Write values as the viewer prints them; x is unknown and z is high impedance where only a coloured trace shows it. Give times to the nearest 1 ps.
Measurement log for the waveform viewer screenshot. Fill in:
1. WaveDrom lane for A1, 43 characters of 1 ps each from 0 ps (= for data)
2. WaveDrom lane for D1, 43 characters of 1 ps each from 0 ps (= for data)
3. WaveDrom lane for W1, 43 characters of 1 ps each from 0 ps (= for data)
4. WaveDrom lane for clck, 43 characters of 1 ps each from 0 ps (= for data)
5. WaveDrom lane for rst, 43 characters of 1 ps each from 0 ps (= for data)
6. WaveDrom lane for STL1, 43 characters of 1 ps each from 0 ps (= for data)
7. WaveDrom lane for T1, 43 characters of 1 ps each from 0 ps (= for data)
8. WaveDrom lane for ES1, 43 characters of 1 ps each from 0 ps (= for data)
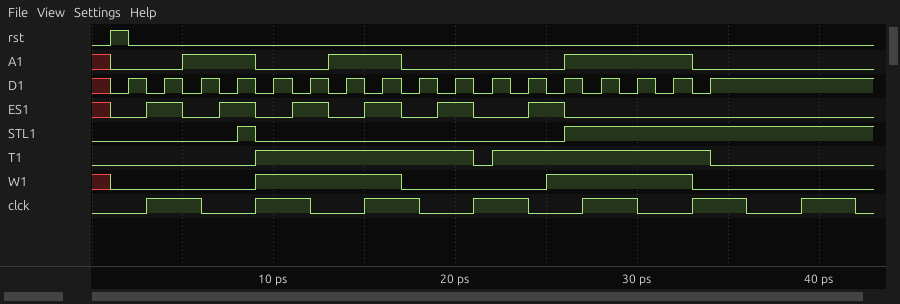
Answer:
{name: 'A1', wave: 'x0...1...0...1...0........1......0.........'}
{name: 'D1', wave: 'x0101010101010101010101010101010101........'}
{name: 'W1', wave: 'x0.......1.......0.......1.......0.........'}
{name: 'clck', wave: '0..1..0..1..0..1..0..1..0..1..0..1..0..1..0'}
{name: 'rst', wave: '010........................................'}
{name: 'STL1', wave: '0.......10................1................'}
{name: 'T1', wave: '0........1...........01...........0........'}
{name: 'ES1', wave: 'x0.1.0.1.0.1.0.1.0.1.0..1.0................'}
